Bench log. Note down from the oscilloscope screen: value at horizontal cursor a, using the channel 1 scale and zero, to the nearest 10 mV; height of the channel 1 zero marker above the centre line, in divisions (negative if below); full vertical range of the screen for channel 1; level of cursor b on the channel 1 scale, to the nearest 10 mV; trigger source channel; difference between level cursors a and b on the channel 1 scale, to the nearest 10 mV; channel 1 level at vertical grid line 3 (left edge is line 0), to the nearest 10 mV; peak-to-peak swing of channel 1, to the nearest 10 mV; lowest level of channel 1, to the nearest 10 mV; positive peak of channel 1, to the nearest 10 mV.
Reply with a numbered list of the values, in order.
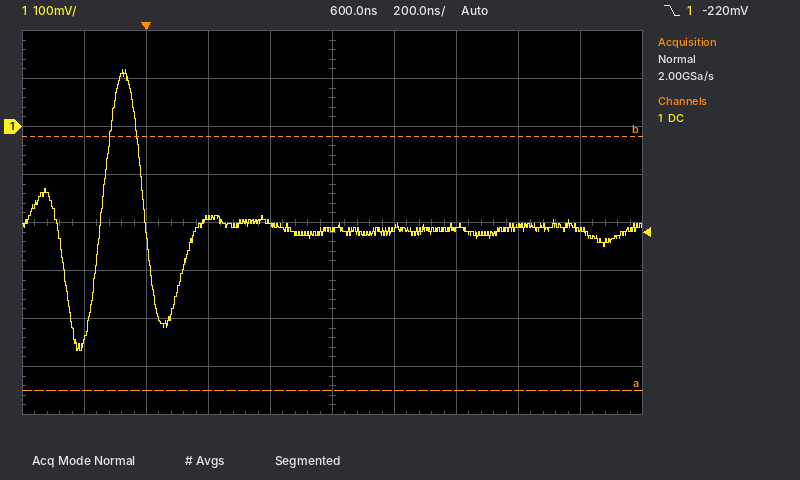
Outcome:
1. -550 mV
2. +2.0 div
3. 800 mV
4. -20 mV
5. channel 1
6. 530 mV
7. -190 mV
8. 590 mV
9. -470 mV
10. 120 mV
